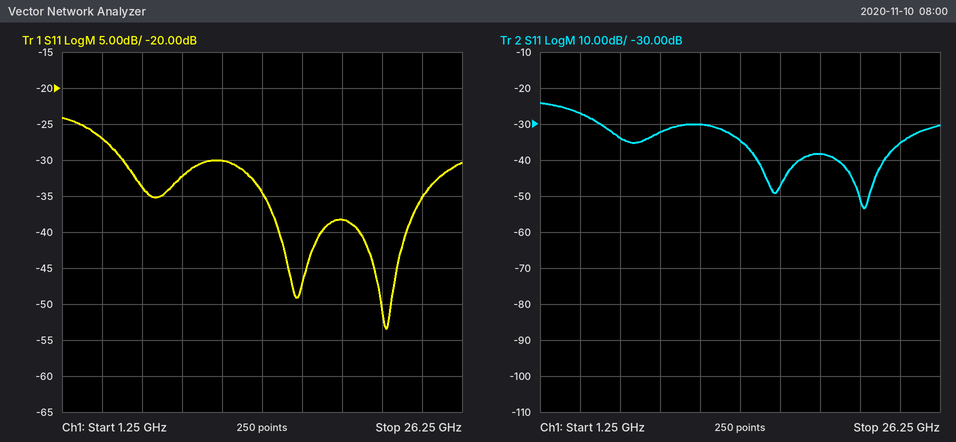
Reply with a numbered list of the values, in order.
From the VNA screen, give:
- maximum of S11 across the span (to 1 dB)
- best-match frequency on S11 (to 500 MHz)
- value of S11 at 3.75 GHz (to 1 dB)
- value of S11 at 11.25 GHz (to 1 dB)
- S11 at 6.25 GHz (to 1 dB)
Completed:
1. -24 dB
2. 21.5 GHz
3. -27 dB
4. -30 dB
5. -34 dB
